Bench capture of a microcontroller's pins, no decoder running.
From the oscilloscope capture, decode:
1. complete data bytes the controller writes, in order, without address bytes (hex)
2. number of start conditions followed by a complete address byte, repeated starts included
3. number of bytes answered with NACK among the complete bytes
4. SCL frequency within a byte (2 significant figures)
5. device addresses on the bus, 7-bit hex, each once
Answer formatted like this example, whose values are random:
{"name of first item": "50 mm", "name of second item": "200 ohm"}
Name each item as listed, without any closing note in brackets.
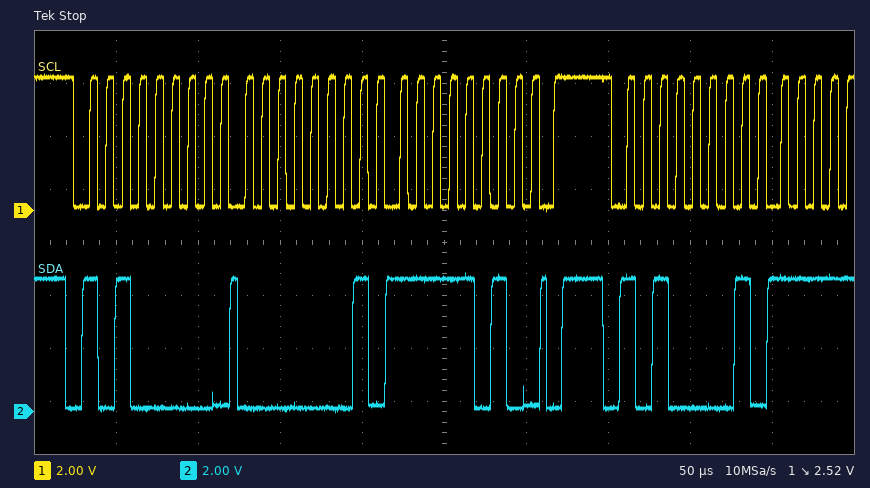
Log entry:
{"complete data bytes the controller writes, in order, without address bytes": "01 FA", "number of start conditions followed by a complete address byte, repeated starts included": "2", "number of bytes answered with NACK among the complete bytes": "0", "SCL frequency within a byte": "100 kHz", "device addresses on the bus, 7-bit hex, each once": "0x50"}
